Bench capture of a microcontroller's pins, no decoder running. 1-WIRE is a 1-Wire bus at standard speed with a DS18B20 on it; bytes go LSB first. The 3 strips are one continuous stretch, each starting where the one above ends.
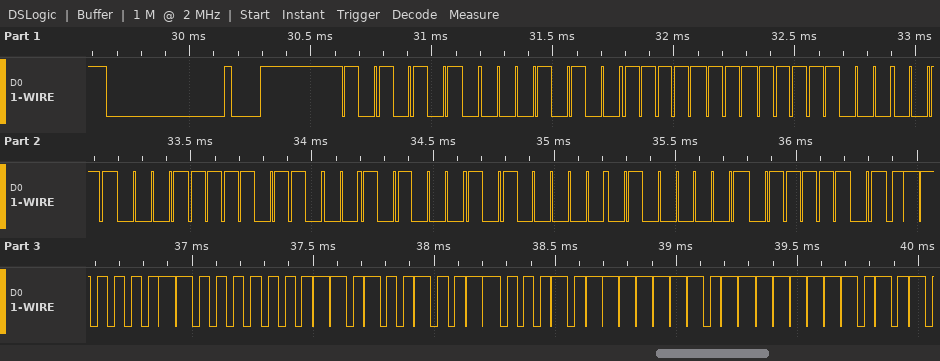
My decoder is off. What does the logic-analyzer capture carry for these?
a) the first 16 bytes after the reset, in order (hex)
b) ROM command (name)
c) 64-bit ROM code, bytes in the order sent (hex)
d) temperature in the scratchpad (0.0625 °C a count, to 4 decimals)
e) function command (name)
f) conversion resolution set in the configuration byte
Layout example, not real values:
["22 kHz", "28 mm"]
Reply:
["55 28 FF 1F 8C 6F 14 05 82 BE 86 01 4B 46 7F FF", "Match ROM", "28 FF 1F 8C 6F 14 05 82", "24.3750 °C", "Read Scratchpad", "12 bits"]
